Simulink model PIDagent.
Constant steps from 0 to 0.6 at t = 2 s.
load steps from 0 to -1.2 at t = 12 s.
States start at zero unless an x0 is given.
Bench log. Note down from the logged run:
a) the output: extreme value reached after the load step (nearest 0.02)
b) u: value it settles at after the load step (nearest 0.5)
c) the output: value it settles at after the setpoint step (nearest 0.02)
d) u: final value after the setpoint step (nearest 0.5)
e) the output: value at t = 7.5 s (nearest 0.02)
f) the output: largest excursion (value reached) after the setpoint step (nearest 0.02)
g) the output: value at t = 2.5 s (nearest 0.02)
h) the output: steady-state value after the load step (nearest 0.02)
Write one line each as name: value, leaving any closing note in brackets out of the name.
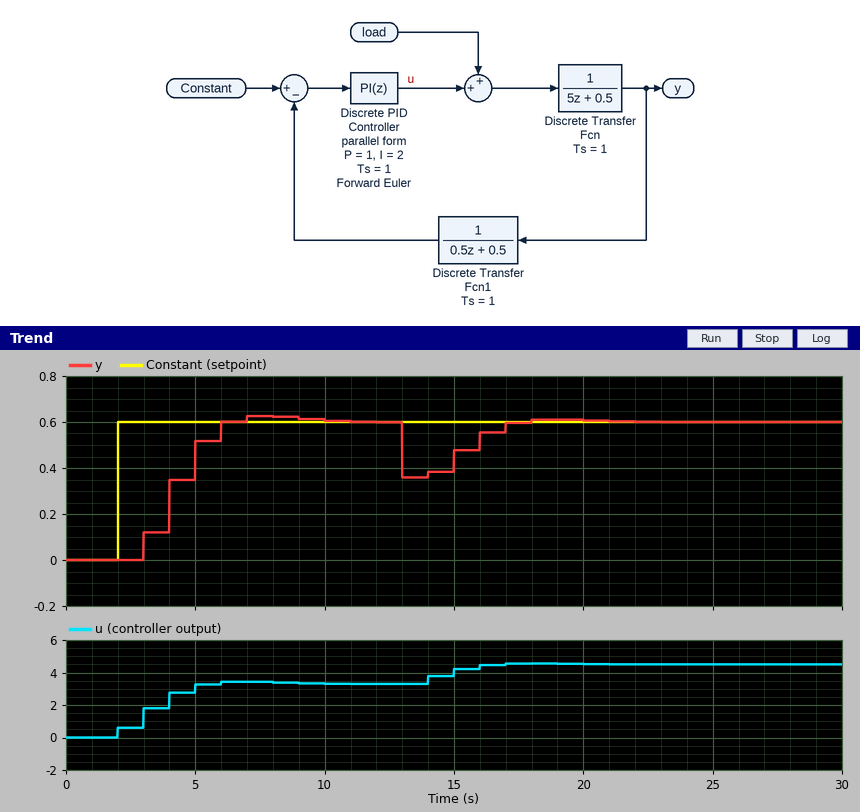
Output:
the output: extreme value reached after the load step: 0.36
u: value it settles at after the load step: 4.5
the output: value it settles at after the setpoint step: 0.60
u: final value after the setpoint step: 3.5
the output: value at t = 7.5 s: 0.62
the output: largest excursion (value reached) after the setpoint step: 0.62
the output: value at t = 2.5 s: 0.00
the output: steady-state value after the load step: 0.60
